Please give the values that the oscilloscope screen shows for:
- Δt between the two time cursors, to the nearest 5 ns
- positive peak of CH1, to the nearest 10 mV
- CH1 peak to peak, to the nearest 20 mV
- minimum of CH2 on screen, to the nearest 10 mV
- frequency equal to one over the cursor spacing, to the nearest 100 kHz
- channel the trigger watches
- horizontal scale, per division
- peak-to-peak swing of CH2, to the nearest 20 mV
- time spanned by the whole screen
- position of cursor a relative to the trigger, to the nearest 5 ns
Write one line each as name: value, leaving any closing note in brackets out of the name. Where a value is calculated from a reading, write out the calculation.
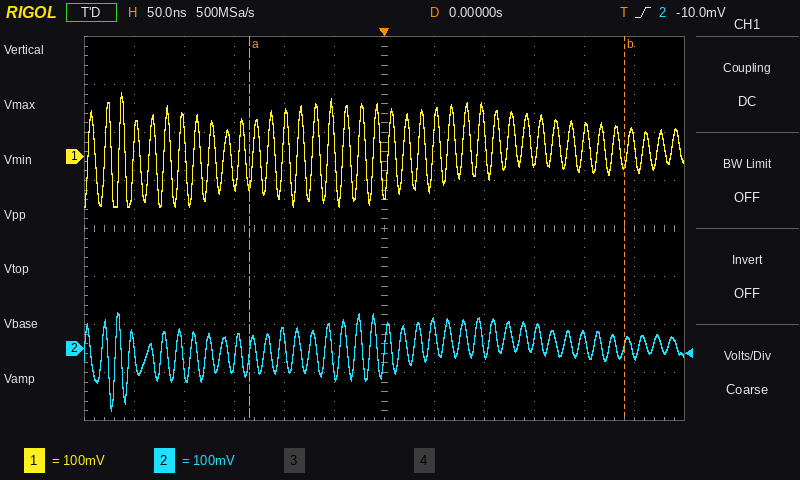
Δt between the two time cursors, to the nearest 5 ns: 375 ns
positive peak of CH1, to the nearest 10 mV: 130 mV
CH1 peak to peak, to the nearest 20 mV: 240 mV
minimum of CH2 on screen, to the nearest 10 mV: -130 mV
frequency equal to one over the cursor spacing, to the nearest 100 kHz: 1 / 375 ns ≈ 2.7 MHz
channel the trigger watches: CH2
horizontal scale, per division: 50 ns
peak-to-peak swing of CH2, to the nearest 20 mV: 200 mV
time spanned by the whole screen: 600 ns
position of cursor a relative to the trigger, to the nearest 5 ns: -135 ns
